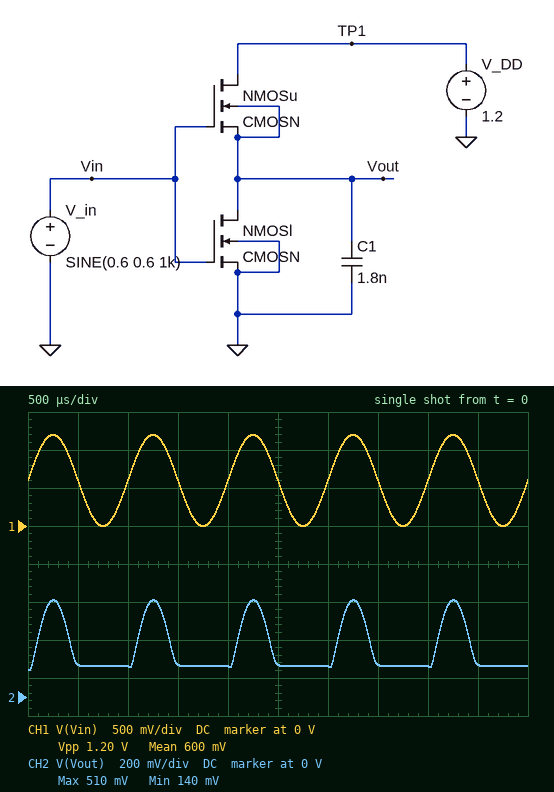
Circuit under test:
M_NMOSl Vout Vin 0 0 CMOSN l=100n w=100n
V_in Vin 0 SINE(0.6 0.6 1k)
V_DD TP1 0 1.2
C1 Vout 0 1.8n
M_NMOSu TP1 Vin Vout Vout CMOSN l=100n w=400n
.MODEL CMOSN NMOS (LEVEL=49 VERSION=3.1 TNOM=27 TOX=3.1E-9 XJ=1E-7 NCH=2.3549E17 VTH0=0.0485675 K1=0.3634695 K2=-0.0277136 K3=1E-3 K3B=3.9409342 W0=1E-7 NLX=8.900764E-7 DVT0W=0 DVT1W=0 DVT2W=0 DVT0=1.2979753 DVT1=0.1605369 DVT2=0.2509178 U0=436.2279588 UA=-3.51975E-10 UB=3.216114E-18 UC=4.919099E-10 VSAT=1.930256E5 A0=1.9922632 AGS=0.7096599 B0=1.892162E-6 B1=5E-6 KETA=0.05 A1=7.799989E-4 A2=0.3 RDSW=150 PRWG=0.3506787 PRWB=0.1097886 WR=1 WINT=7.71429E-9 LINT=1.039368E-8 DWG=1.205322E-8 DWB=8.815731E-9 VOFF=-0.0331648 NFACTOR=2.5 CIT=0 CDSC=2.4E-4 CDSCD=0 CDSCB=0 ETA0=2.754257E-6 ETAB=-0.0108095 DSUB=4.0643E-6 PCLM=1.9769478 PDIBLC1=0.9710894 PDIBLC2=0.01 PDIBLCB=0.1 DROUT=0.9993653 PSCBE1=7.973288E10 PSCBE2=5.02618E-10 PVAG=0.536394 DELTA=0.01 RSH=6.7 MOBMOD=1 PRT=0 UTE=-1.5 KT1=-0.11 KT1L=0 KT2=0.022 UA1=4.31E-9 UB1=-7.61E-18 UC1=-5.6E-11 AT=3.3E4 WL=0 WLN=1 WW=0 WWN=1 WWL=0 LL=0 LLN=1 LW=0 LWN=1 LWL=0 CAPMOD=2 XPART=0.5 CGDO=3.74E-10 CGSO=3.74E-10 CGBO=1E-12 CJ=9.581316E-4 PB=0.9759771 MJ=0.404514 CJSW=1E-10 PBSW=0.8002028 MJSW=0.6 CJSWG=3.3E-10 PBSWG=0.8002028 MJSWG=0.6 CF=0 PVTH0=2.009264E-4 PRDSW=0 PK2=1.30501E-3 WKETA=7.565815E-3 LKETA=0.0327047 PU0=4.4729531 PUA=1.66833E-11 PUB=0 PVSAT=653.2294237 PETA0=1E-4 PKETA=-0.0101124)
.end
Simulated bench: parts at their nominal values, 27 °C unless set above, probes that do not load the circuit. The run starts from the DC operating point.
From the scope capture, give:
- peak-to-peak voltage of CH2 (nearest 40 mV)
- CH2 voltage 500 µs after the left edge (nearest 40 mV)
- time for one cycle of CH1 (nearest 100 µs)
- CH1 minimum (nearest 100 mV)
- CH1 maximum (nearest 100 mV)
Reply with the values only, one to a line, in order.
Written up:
360 mV
160 mV
1.0 ms
0 V
1.2 V
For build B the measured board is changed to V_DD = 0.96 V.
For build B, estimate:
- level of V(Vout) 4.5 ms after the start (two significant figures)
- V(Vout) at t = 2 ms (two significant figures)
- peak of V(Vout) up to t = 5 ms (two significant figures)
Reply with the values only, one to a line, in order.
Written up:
160 mV
150 mV
490 mV
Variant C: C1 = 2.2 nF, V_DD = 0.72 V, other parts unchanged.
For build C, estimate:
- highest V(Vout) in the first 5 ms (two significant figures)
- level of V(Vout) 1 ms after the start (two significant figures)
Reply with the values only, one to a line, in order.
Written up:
460 mV
150 mV
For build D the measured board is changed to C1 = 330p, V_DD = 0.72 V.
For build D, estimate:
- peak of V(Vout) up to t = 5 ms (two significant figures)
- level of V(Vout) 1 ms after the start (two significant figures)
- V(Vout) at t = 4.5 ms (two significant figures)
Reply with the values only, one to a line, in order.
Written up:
460 mV
120 mV
130 mV
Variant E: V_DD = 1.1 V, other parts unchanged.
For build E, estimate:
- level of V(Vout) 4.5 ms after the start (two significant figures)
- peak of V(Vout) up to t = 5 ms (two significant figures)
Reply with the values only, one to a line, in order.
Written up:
160 mV
500 mV
